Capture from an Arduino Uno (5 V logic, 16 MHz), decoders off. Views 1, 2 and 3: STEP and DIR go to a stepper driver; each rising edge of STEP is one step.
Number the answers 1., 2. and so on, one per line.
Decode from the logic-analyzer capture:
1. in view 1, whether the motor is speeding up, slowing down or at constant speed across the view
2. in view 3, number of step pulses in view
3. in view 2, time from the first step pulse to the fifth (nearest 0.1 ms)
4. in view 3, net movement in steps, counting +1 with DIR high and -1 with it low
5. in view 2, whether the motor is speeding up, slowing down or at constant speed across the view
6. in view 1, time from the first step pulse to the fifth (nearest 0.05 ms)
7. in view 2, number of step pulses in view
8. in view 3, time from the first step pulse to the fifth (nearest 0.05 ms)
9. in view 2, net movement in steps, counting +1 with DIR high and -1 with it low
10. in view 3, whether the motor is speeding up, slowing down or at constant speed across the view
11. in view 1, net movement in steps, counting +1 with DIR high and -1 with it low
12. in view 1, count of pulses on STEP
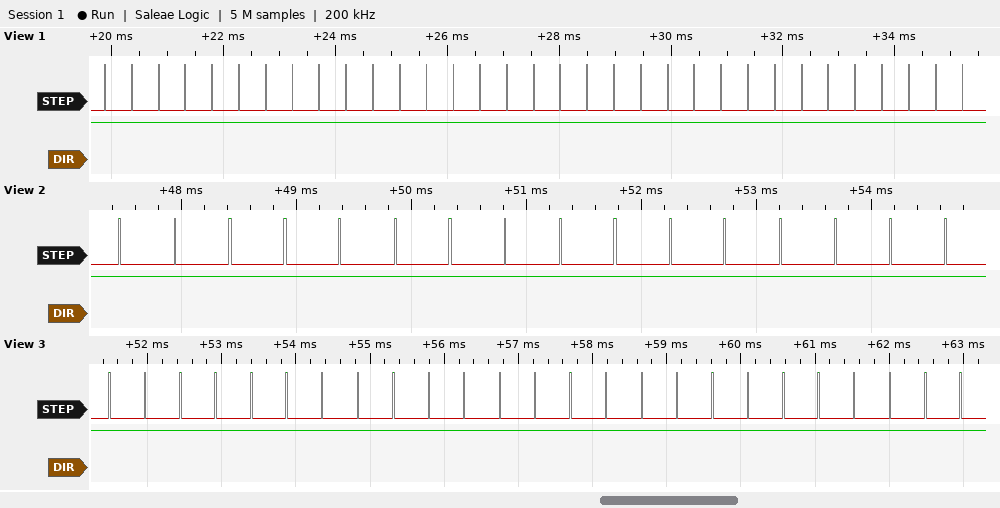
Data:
1. constant speed
2. 25
3. 1.9 ms
4. +25
5. constant speed
6. 1.90 ms
7. 16
8. 1.90 ms
9. +16
10. constant speed
11. +33
12. 33
